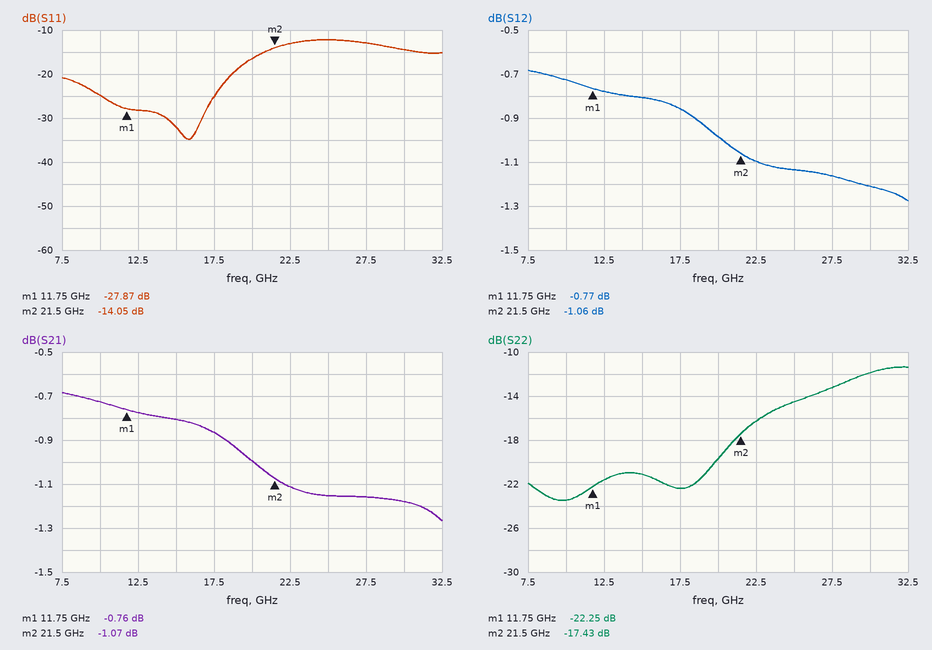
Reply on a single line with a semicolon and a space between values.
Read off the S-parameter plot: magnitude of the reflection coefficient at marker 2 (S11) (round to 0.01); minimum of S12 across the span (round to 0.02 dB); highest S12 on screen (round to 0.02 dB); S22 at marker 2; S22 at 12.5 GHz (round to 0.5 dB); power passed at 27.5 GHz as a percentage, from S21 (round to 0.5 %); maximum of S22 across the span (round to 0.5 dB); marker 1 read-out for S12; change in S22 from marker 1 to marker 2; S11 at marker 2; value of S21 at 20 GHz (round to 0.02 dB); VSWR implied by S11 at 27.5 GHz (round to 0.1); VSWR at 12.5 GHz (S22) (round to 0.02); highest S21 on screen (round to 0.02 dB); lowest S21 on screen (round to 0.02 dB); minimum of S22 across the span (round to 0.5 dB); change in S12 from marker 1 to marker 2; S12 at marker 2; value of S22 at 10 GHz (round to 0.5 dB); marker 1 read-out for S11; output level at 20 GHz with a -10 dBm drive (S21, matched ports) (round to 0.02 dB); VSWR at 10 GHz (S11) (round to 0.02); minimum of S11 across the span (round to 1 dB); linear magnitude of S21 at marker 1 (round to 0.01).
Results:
0.20; -1.28 dB; -0.68 dB; -17.43 dB; -21.5 dB; 76.5 %; -11.5 dB; -0.77 dB; 4.82 dB; -14.05 dB; -1.00 dB; 1.6; 1.18; -0.68 dB; -1.26 dB; -23.5 dB; -0.29 dB; -1.06 dB; -23.5 dB; -27.87 dB; -11.00 dBm; 1.12; -35 dB; 0.92
